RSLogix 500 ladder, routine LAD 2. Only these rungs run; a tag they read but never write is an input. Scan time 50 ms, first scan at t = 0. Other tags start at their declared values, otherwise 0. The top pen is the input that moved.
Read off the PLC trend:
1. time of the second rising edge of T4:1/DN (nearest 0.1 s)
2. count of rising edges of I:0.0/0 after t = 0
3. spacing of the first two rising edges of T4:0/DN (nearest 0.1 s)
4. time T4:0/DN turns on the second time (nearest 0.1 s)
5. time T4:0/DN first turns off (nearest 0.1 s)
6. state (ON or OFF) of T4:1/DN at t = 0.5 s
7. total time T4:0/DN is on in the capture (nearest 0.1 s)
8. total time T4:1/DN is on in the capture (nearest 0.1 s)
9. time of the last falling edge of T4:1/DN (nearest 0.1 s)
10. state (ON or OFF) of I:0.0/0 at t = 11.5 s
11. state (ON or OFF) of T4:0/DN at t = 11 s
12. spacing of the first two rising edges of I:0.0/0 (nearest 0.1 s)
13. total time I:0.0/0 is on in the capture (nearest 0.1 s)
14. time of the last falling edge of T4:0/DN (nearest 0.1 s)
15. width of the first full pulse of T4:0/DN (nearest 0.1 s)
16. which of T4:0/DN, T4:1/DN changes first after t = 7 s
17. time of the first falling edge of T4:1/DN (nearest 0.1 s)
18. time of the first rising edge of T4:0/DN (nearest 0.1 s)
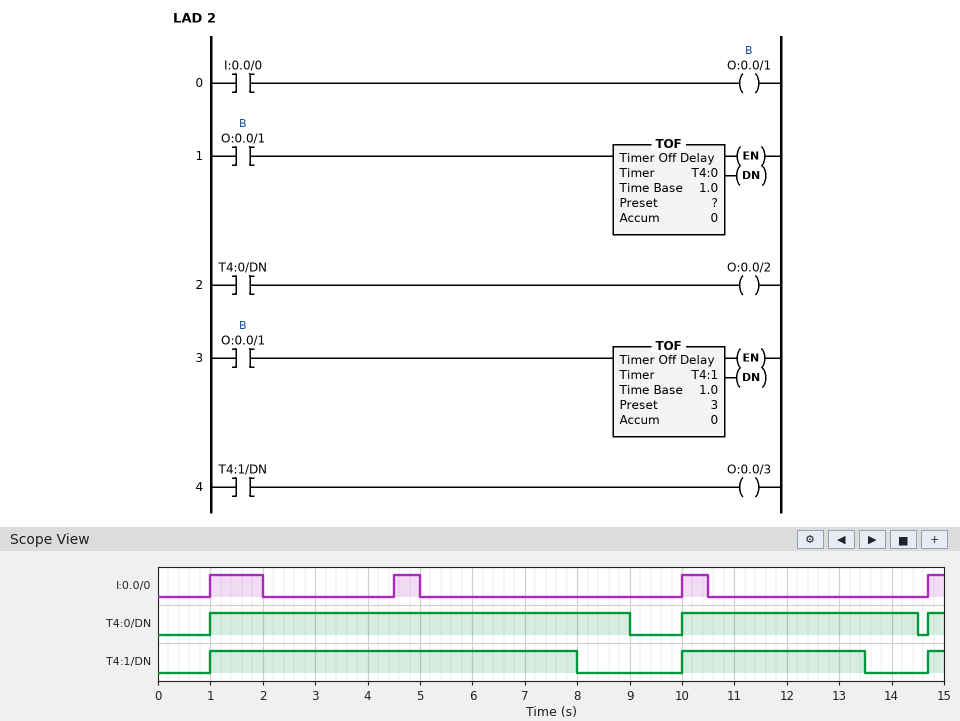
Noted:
10.0 s
4
9.0 s
10.0 s
9.0 s
OFF
12.8 s
10.8 s
13.5 s
OFF
ON
3.5 s
2.3 s
14.5 s
8.0 s
T4:1/DN
8.0 s
1.0 s
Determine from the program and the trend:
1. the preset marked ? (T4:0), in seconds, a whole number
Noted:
4 s
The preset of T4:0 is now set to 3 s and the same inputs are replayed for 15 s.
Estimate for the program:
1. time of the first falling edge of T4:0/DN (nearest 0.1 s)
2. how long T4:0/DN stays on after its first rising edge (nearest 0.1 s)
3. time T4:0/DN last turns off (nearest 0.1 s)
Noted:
8.0 s
7.0 s
13.5 s
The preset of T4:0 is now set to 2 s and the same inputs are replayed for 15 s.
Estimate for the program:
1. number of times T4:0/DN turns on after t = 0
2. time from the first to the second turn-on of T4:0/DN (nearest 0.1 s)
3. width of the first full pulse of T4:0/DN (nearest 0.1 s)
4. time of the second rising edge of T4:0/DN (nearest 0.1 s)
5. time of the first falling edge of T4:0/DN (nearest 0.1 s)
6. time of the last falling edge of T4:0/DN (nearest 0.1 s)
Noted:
4
3.5 s
3.0 s
4.5 s
4.0 s
12.5 s
